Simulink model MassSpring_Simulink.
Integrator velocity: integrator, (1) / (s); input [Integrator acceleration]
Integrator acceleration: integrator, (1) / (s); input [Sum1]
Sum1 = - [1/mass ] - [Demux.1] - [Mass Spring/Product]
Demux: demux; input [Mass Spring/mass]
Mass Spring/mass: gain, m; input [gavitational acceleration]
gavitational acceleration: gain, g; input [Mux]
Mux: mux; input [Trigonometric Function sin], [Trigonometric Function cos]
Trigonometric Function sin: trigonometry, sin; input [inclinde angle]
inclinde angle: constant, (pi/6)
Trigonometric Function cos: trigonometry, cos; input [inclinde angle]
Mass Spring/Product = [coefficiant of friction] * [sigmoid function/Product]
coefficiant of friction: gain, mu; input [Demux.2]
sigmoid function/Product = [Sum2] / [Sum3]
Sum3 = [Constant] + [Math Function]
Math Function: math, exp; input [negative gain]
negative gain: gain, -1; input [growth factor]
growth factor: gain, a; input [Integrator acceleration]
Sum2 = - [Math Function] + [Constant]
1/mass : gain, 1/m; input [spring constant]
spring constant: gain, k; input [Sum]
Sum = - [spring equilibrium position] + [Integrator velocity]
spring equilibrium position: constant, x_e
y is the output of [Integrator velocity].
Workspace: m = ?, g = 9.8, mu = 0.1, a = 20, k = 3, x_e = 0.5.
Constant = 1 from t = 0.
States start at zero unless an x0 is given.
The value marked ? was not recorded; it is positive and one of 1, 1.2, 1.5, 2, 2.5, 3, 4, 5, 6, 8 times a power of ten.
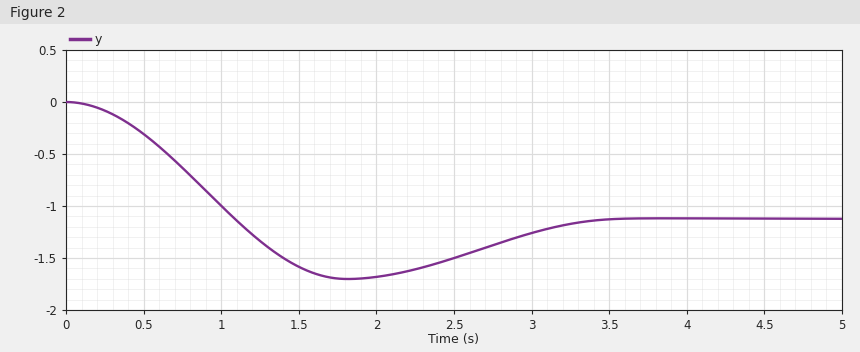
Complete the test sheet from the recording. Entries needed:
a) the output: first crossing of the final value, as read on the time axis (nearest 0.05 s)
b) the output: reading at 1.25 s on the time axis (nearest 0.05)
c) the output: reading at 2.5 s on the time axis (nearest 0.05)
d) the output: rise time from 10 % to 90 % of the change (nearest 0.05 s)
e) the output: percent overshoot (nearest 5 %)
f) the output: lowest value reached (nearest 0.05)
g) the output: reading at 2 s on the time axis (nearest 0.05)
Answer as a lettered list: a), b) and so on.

a) 1.10 s
b) -1.35
c) -1.50
d) 0.70 s
e) 50 %
f) -1.70
g) -1.70
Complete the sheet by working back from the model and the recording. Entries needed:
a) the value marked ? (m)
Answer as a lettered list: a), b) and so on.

a) 1
